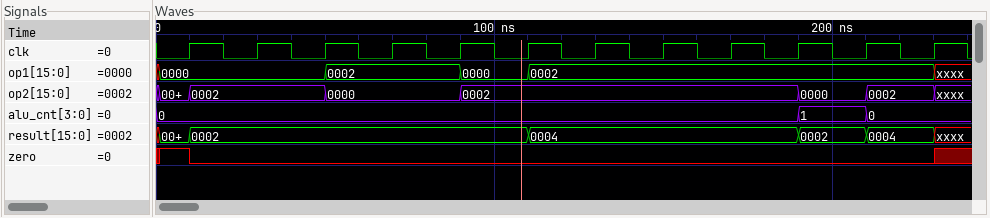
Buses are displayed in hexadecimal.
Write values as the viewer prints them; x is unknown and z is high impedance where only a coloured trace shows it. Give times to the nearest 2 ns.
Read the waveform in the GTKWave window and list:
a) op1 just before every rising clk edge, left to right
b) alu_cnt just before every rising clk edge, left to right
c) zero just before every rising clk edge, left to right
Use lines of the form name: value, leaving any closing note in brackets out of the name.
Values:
op1 just before every rising clk edge, left to right: 0000, 0000, 0000, 0002, 0002, 0000, 0002, 0002, 0002, 0002, 0002, 0002
alu_cnt just before every rising clk edge, left to right: 0, 0, 0, 0, 0, 0, 0, 0, 0, 0, 1, 0
zero just before every rising clk edge, left to right: 1 0 0 0 0 0 0 0 0 0 0 0
